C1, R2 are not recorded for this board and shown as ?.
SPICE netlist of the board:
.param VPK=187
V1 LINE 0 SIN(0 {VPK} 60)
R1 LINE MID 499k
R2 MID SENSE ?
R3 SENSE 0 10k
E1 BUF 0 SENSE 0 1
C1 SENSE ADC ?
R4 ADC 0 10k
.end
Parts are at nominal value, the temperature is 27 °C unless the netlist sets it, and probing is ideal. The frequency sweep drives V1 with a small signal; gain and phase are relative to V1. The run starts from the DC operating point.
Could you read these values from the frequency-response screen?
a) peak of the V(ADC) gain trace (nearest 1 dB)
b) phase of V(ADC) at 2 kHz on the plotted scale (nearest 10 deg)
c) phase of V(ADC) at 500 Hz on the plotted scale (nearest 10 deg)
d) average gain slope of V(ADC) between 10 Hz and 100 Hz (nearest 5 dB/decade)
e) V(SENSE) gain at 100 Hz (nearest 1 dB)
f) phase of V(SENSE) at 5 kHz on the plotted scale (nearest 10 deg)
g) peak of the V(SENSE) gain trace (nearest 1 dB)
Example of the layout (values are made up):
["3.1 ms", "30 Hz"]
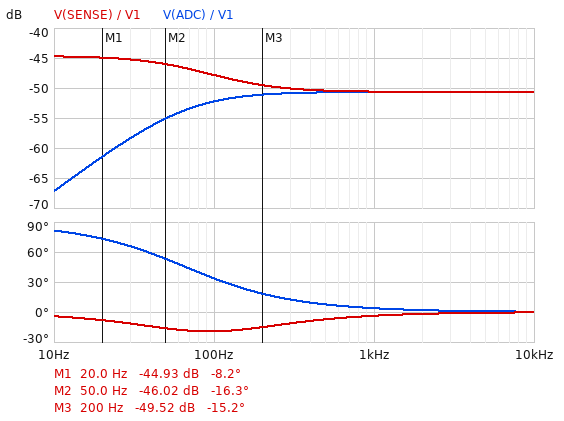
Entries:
["-51 dB", "0 deg", "10 deg", "15 dB/decade", "-48 dB", "0 deg", "-45 dB"]
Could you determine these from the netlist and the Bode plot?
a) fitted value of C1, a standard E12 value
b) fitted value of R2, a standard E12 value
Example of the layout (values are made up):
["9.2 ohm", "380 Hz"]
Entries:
["120 nF", "1.2 MΩ"]
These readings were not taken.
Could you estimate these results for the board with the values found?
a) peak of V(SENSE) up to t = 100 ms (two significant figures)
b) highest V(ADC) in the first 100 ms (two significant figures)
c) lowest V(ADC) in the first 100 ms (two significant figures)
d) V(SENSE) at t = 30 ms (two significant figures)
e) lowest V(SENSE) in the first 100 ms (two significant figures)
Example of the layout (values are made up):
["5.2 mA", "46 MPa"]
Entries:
["930 mV", "370 mV", "-370 mV", "-890 mV", "-890 mV"]
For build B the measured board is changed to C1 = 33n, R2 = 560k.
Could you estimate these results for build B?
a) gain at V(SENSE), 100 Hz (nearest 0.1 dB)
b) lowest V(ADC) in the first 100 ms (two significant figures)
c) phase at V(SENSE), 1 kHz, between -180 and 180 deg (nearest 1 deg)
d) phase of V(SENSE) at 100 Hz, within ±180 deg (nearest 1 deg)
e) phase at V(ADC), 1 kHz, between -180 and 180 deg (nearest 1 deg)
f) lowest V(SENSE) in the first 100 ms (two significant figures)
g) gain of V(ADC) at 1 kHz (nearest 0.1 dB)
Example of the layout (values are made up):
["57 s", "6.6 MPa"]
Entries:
["-41.1 dB", "-210 mV", "-12 deg", "-11 deg", "14 deg", "-1.7 V", "-46.8 dB"]
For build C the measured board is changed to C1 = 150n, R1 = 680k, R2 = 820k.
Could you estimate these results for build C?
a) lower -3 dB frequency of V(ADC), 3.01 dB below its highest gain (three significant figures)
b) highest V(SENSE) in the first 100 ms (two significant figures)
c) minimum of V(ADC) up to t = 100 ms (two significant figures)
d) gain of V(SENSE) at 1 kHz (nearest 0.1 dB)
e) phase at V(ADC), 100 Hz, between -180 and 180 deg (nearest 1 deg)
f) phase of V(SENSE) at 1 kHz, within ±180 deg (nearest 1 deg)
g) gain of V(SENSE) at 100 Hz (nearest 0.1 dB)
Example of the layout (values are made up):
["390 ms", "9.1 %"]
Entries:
["53.2 Hz", "1.0 V", "-470 mV", "-49.5 dB", "28 deg", "-3 deg", "-47.4 dB"]
